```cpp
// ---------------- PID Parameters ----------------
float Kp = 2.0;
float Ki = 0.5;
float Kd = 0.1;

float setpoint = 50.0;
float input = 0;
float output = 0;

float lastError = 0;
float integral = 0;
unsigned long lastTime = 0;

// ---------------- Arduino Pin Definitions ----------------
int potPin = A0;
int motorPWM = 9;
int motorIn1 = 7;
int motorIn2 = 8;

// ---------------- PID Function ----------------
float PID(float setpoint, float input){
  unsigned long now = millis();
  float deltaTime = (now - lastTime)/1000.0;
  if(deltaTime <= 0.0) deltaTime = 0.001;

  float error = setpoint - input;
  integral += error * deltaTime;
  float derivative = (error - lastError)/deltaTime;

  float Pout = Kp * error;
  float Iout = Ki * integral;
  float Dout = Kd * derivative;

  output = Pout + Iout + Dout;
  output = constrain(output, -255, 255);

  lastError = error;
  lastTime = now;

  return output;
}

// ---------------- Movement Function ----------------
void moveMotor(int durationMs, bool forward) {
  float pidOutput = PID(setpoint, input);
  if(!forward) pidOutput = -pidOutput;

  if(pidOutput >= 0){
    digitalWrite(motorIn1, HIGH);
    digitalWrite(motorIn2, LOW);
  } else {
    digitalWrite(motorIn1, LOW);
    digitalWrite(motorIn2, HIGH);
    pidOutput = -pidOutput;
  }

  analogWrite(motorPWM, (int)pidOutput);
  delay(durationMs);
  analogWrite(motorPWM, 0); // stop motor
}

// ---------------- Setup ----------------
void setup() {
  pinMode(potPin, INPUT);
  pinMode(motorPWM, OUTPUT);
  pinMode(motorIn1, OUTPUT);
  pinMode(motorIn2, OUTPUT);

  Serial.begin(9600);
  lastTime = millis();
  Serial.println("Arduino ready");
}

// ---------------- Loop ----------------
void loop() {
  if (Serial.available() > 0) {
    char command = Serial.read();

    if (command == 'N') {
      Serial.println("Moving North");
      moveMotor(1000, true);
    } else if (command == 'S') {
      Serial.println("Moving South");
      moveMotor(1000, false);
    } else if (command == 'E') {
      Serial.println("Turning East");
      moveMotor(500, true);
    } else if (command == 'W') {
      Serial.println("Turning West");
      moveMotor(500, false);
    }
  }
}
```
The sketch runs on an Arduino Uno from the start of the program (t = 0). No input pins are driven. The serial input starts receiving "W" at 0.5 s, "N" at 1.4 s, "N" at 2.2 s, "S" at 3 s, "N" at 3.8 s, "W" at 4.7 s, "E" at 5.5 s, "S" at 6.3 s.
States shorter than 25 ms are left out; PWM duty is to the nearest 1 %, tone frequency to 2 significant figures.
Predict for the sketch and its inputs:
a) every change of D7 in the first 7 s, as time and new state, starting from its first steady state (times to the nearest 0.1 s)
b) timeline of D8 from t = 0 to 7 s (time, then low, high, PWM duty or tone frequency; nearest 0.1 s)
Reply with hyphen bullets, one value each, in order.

- 0 s low; 1.4 s high; 3.4 s low; 4.4 s high; 5.4 s low; 5.9 s high; 6.4 s low
- 0 s low; 0.5 s high; 1.4 s low; 3.4 s high; 4.4 s low; 5.4 s high; 5.9 s low; 6.4 s high
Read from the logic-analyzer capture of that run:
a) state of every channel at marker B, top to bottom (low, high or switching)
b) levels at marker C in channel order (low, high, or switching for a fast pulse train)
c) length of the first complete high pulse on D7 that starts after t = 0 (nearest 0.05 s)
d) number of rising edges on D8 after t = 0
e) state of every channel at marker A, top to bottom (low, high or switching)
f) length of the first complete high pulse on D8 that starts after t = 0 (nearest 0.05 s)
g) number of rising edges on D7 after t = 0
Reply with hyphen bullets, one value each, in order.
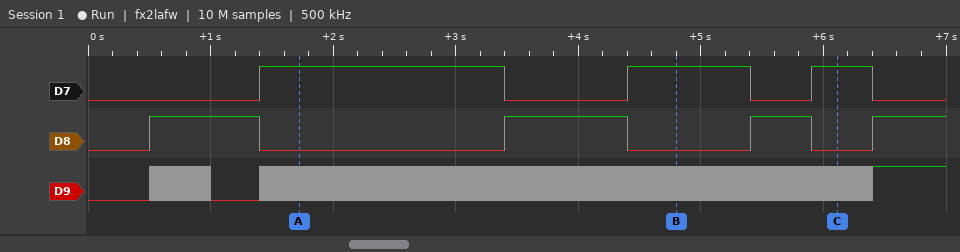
- D7 high, D8 low, D9 switching
- D7 high, D8 low, D9 switching
- 2.00 s
- 4
- D7 high, D8 low, D9 switching
- 0.90 s
- 3
